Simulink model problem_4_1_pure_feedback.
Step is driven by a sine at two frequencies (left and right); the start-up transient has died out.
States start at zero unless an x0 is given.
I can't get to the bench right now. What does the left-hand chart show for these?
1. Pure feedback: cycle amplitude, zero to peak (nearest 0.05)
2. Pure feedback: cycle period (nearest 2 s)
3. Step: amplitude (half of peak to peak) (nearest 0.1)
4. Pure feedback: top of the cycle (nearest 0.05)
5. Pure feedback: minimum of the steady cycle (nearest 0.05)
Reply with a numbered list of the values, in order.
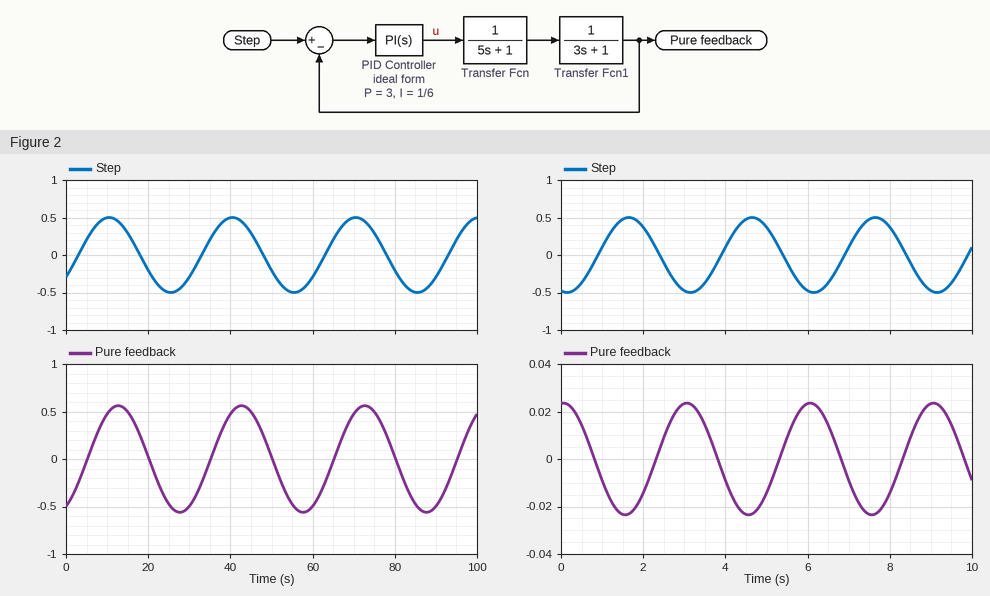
1. 0.55
2. 30 s
3. 0.5
4. 0.55
5. -0.55
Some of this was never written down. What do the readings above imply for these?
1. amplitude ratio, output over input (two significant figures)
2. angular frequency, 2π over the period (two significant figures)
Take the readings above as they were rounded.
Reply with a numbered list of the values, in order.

1. 1.1
2. 0.21 rad/s
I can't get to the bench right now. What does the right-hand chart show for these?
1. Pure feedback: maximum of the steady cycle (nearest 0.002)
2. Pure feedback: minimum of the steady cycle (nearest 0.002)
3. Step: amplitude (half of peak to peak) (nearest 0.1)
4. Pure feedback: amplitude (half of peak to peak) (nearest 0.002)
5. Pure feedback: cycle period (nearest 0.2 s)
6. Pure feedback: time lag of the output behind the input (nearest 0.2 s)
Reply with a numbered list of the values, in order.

1. 0.024
2. -0.024
3. 0.5
4. 0.024
5. 3.0 s
6. 1.4 s
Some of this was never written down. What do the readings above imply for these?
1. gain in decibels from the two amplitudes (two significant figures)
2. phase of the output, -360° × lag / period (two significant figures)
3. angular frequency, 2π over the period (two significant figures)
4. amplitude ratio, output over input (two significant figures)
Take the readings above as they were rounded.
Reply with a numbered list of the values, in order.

1. -26 dB
2. -170°
3. 2.1 rad/s
4. 0.048
